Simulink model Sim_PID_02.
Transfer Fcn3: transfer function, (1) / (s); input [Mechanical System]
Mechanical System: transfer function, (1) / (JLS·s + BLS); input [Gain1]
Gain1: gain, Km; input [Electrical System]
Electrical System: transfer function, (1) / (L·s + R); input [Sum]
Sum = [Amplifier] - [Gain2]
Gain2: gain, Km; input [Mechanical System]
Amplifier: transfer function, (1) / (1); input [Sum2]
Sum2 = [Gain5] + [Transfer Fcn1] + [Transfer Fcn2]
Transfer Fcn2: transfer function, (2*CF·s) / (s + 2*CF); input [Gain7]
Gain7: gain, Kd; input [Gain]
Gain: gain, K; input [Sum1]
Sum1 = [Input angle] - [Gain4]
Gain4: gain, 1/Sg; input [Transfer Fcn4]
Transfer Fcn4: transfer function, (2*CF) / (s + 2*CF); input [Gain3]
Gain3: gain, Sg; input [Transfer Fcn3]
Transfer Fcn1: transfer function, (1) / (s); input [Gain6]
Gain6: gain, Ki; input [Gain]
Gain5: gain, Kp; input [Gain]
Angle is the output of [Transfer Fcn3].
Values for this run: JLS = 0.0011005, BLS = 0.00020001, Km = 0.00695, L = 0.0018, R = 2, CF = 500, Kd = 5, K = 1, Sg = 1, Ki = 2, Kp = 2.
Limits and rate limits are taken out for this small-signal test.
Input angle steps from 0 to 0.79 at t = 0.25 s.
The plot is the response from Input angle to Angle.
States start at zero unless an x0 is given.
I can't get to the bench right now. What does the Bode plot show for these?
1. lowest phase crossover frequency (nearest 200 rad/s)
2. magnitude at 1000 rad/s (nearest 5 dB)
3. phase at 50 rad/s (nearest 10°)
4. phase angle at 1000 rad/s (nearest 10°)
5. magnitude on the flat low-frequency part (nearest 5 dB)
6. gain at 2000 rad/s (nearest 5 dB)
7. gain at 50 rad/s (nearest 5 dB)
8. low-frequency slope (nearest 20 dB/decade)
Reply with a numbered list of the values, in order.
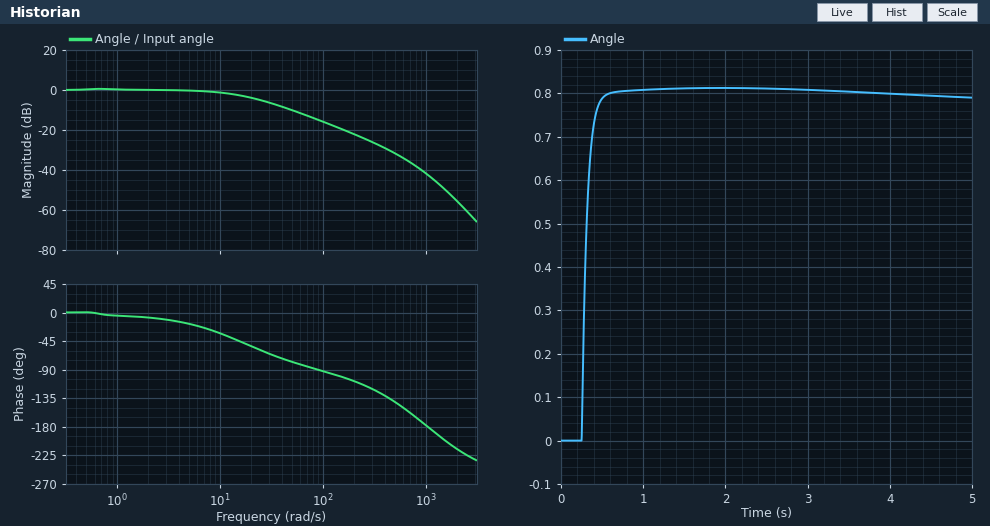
1. 1000 rad/s
2. -40 dB
3. -80°
4. -180°
5. 0 dB
6. -55 dB
7. -10 dB
8. 0 dB/decade
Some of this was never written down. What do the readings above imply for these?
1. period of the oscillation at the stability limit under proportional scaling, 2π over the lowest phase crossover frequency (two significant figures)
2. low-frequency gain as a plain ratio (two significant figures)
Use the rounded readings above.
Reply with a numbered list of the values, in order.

1. 0.0063 s
2. 1.0
